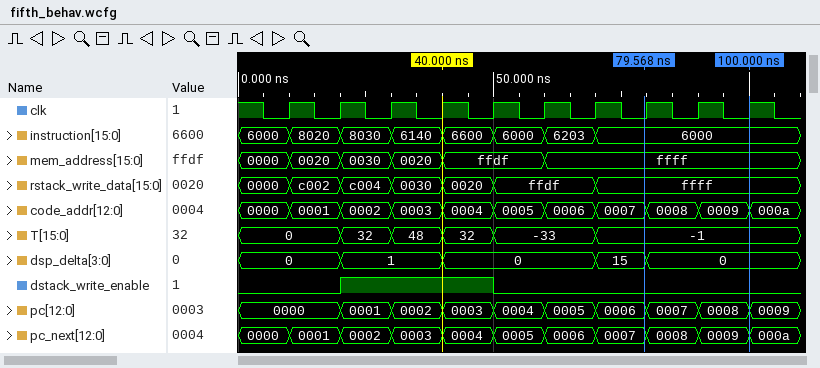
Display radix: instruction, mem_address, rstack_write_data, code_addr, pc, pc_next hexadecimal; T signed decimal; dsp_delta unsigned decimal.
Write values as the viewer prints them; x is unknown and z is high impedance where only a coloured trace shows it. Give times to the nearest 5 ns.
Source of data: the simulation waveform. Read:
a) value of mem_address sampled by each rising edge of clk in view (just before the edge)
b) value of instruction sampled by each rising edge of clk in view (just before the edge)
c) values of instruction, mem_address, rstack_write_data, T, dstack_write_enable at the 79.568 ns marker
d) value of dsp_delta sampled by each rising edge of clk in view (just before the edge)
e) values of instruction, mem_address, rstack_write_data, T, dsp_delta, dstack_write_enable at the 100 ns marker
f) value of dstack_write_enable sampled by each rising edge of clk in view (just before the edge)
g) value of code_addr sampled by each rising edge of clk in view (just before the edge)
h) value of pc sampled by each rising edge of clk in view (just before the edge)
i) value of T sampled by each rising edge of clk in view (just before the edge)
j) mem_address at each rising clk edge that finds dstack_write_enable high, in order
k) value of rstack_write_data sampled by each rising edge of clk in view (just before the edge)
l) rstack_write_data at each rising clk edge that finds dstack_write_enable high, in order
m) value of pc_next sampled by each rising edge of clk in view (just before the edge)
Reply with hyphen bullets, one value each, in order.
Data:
- 0000, 0020, 0030, 0020, ffdf, ffdf, ffff, ffff, ffff, ffff
- 6000, 8020, 8030, 6140, 6600, 6000, 6203, 6000, 6000, 6000
- instruction=6000, mem_address=ffff, rstack_write_data=ffff, T=-1, dstack_write_enable=0
- 0, 0, 1, 1, 0, 0, 0, 15, 0, 0
- instruction=6000, mem_address=ffff, rstack_write_data=ffff, T=-1, dsp_delta=0, dstack_write_enable=0
- 0 0 1 1 1 0 0 0 0 0
- 0000, 0001, 0002, 0003, 0004, 0005, 0006, 0007, 0008, 0009
- 0000, 0000, 0001, 0002, 0003, 0004, 0005, 0006, 0007, 0008
- 0, 0, 32, 48, 32, -33, -33, -1, -1, -1
- 0030, 0020, ffdf
- 0000, c002, c004, 0030, 0020, ffdf, ffdf, ffff, ffff, ffff
- c004, 0030, 0020
- 0000, 0001, 0002, 0003, 0004, 0005, 0006, 0007, 0008, 0009
